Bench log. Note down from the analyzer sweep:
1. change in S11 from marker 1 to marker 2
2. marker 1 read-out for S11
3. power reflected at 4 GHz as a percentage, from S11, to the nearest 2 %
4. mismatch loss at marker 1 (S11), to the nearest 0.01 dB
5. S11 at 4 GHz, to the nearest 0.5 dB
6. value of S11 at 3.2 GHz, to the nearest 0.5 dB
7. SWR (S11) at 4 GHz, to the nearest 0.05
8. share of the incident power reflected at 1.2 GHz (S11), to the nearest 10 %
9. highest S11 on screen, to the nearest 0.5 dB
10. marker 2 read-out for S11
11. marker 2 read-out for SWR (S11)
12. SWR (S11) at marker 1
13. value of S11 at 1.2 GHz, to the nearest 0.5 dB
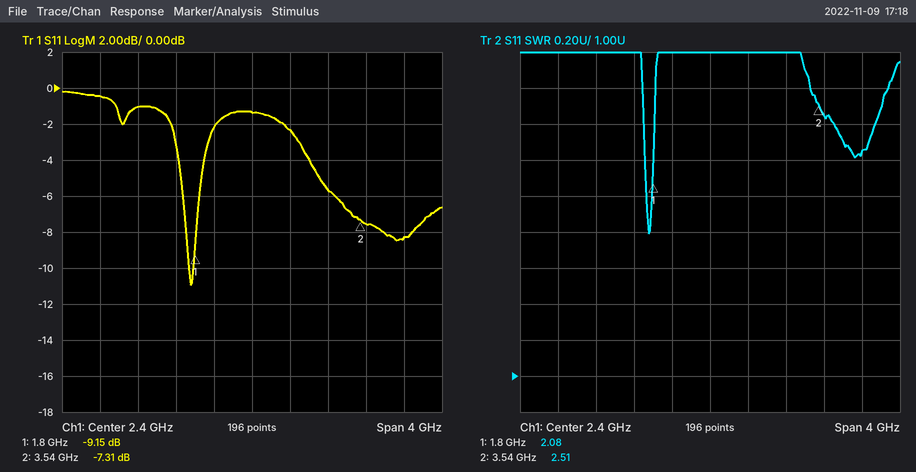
1.84 dB
-9.15 dB
14 %
0.56 dB
-8.5 dB
-5.5 dB
2.25
80 %
0.0 dB
-7.31 dB
2.51
2.08
-1.0 dB
